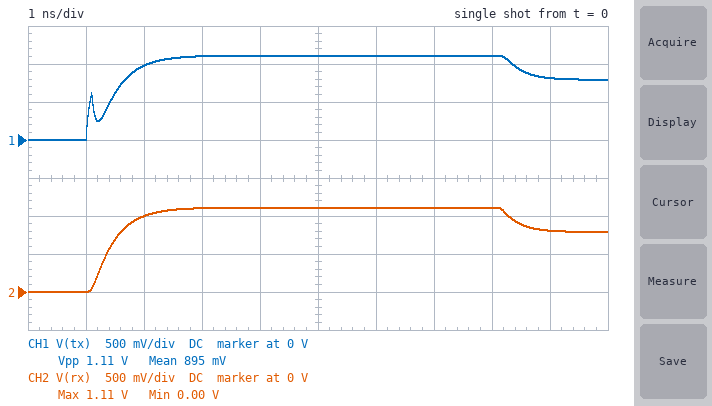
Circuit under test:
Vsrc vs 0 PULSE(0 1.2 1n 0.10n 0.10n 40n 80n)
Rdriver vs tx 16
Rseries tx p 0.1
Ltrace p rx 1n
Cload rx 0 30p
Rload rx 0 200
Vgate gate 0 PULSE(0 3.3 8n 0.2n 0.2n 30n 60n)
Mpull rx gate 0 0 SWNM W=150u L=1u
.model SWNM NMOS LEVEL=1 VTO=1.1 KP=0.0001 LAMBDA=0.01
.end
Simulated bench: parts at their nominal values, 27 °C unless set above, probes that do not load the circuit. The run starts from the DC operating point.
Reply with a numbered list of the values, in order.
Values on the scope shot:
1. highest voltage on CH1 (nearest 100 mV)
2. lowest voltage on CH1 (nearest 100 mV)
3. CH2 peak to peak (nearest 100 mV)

1. 1.1 V
2. 0 V
3. 1.1 V
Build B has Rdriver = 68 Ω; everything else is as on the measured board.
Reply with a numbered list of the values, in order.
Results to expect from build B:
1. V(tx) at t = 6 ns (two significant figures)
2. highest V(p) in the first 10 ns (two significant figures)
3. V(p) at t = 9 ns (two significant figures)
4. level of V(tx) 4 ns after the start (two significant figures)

1. 860 mV
2. 890 mV
3. 500 mV
4. 770 mV
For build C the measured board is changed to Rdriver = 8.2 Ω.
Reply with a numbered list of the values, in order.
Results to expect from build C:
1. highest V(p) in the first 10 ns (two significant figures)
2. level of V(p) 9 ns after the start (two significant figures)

1. 1.2 V
2. 950 mV
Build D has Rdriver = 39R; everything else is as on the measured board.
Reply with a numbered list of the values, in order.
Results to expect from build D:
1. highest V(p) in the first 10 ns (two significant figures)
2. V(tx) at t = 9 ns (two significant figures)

1. 1.0 V
2. 620 mV
